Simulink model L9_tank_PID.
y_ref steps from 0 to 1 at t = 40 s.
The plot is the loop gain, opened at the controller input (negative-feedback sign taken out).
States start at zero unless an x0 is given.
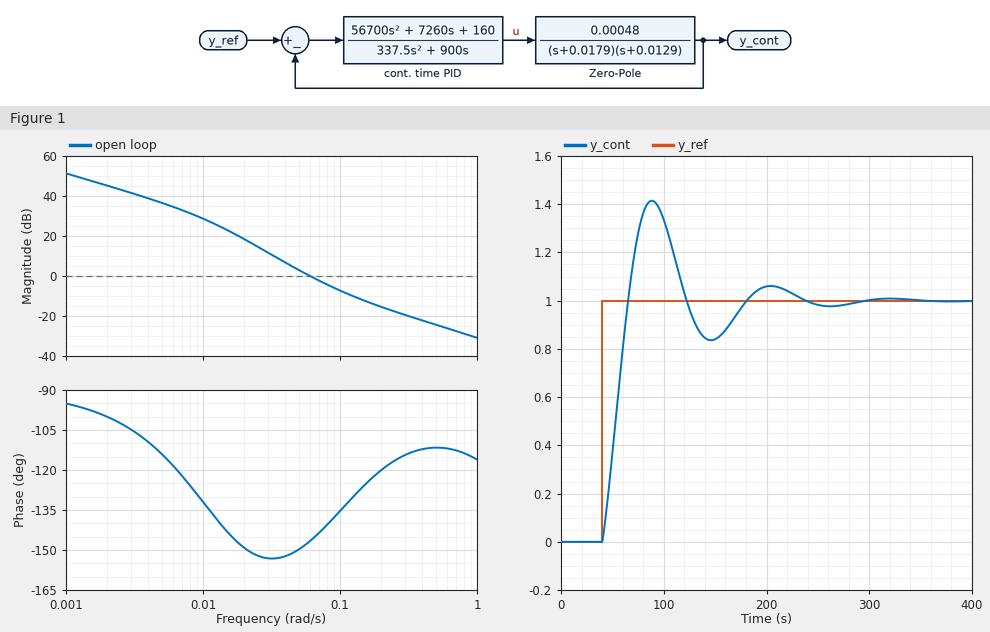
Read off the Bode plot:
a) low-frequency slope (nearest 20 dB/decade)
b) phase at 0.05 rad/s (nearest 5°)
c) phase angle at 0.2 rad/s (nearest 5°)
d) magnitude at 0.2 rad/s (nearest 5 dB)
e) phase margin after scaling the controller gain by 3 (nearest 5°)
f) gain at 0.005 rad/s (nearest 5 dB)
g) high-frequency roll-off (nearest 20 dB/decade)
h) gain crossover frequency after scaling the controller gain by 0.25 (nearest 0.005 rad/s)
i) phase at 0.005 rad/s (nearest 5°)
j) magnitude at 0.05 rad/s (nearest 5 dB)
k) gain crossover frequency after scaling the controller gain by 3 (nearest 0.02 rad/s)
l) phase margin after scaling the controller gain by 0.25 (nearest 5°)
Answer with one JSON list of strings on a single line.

["-20 dB/decade", "-150°", "-120°", "-15 dB", "50°", "35 dB", "-20 dB/decade", "0.030 rad/s", "-115°", "5 dB", "0.12 rad/s", "25°"]
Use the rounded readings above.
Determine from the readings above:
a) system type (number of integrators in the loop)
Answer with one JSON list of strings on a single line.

["1"]
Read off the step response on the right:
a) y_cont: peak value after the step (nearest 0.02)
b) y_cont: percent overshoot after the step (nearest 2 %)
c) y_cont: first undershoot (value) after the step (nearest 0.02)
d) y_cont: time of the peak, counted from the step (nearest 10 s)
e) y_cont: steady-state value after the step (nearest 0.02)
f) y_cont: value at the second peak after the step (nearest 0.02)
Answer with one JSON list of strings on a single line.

["1.42", "42 %", "0.84", "50 s", "1.00", "1.06"]
